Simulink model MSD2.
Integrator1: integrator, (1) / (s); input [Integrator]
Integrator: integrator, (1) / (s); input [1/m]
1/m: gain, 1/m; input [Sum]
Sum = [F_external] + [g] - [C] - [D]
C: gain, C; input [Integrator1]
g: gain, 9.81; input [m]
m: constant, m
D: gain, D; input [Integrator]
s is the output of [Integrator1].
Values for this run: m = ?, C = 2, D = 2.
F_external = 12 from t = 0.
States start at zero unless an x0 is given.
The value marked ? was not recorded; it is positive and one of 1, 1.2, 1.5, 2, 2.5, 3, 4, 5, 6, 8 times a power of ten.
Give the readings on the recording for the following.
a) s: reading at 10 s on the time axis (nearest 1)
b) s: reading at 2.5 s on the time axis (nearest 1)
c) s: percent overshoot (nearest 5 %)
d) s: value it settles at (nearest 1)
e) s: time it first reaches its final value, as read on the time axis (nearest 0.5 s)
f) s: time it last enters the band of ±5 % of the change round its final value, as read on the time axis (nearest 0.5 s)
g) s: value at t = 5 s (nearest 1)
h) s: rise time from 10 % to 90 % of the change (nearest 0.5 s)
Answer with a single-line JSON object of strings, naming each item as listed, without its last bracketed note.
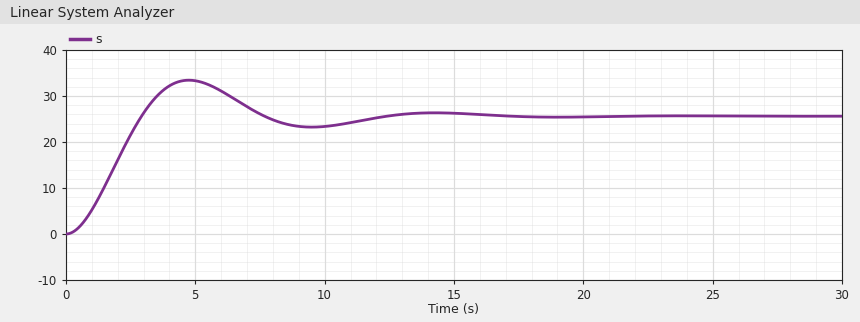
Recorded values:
{"s: reading at 10 s on the time axis": "23", "s: reading at 2.5 s on the time axis": "22", "s: percent overshoot": "30 %", "s: value it settles at": "26", "s: time it first reaches its final value, as read on the time axis": "3.0 s", "s: time it last enters the band of ±5 % of the change round its final value, as read on the time axis": "11.0 s", "s: value at t = 5 s": "33", "s: rise time from 10 % to 90 % of the change": "2.0 s"}
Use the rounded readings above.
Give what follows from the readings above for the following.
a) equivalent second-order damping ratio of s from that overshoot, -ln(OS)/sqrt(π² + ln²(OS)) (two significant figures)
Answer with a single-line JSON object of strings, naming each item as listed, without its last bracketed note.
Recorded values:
{"equivalent second-order damping ratio of s from that overshoot, -ln(OS)/sqrt(π² + ln²(OS))": "0.36"}
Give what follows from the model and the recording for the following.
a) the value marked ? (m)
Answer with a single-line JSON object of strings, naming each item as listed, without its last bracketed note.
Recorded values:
{"the value marked ?": "4"}
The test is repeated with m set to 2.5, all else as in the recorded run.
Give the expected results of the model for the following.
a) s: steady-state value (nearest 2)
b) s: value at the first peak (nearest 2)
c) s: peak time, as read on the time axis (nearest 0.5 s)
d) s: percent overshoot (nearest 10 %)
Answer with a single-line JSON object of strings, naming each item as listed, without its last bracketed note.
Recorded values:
{"s: steady-state value": "18", "s: value at the first peak": "22", "s: peak time, as read on the time axis": "4.0 s", "s: percent overshoot": "20 %"}
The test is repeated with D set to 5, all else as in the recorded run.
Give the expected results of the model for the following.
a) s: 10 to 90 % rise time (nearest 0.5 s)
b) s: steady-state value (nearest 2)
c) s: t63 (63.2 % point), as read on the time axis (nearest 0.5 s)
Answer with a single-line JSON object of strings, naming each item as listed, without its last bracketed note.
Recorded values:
{"s: 10 to 90 % rise time": "4.0 s", "s: steady-state value": "26", "s: t63 (63.2 % point), as read on the time axis": "3.0 s"}
